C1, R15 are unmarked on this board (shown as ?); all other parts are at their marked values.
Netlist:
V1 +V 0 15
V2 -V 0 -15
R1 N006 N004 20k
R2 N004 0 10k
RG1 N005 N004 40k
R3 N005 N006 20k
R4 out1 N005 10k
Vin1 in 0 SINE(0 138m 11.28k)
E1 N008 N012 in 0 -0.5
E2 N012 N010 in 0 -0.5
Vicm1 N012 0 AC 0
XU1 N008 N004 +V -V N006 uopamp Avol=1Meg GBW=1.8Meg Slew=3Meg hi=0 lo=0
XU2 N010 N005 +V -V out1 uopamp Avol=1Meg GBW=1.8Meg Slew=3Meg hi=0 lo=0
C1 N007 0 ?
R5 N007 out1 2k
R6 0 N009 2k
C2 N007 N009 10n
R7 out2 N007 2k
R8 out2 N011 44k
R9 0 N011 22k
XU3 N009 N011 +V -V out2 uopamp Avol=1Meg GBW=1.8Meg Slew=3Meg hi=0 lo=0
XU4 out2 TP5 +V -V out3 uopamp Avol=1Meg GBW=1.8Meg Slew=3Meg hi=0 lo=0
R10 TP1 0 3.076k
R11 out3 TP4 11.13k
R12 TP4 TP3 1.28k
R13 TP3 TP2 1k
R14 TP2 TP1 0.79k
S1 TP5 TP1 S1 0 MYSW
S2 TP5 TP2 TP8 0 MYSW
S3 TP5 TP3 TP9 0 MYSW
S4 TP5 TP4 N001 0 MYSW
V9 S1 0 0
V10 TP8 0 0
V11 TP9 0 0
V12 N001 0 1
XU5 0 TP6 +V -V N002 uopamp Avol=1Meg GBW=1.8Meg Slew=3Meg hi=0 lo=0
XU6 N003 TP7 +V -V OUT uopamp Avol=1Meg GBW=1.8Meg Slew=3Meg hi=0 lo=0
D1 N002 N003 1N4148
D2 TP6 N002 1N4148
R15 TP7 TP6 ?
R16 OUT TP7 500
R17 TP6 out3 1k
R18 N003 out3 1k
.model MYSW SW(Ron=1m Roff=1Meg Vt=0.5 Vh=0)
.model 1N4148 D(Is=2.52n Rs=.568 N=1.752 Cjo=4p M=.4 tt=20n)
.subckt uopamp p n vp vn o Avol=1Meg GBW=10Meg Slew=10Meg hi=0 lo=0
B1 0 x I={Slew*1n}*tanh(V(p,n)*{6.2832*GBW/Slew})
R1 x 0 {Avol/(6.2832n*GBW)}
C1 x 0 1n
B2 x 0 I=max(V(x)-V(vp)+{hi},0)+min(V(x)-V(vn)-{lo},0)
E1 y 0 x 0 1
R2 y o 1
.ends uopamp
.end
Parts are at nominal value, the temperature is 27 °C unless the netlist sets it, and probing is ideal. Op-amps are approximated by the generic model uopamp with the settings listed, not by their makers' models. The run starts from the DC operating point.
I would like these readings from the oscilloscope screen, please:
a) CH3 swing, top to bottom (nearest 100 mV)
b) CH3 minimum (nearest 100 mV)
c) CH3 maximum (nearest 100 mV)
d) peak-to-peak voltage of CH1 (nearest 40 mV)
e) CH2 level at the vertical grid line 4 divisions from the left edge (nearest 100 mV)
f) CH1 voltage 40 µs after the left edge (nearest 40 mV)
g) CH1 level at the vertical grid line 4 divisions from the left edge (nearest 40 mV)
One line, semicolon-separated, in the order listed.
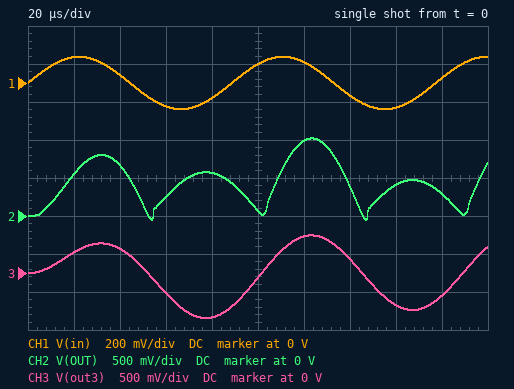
1.1 V; -600 mV; 500 mV; 280 mV; 600 mV; 40 mV; -80 mV
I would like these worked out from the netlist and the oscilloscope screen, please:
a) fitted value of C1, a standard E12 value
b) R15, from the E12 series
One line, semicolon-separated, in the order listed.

33 nF; 470 Ω
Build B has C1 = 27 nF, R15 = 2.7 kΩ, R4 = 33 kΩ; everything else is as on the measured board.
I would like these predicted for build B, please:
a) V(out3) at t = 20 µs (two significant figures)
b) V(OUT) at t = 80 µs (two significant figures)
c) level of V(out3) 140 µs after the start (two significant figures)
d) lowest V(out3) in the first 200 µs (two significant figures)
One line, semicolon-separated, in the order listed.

880 mV; 6.3 V; 610 mV; -2.0 V
